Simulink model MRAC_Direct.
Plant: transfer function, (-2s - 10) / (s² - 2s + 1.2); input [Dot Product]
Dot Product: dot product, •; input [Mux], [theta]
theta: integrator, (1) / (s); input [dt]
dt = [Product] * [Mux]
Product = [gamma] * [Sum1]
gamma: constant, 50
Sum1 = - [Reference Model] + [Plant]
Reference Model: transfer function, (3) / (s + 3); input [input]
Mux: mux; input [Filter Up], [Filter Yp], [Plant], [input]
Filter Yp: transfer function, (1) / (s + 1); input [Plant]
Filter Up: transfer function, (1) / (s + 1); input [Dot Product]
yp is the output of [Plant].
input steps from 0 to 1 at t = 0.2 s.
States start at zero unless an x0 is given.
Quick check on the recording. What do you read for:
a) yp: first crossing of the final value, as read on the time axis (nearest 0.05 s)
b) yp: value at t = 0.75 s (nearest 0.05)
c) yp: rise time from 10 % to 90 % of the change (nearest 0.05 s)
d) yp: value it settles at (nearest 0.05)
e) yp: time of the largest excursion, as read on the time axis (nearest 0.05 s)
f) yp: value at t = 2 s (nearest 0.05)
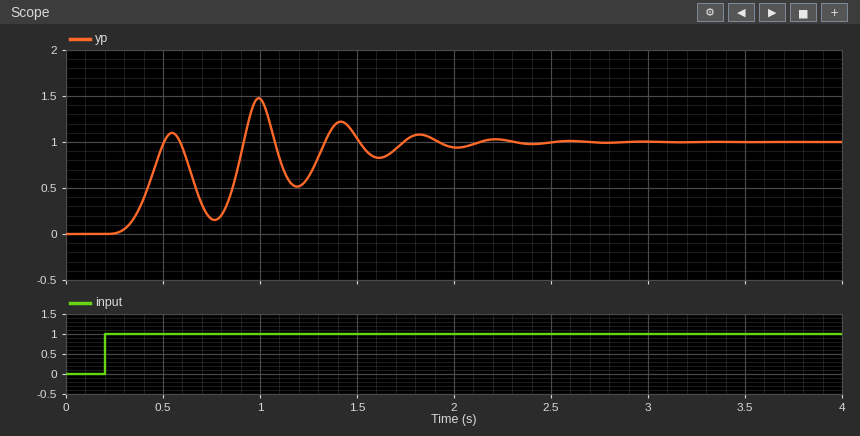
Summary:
0.50 s
0.15
0.15 s
1.00
1.00 s
0.95
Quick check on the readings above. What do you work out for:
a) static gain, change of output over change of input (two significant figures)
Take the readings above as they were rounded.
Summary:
1.0
